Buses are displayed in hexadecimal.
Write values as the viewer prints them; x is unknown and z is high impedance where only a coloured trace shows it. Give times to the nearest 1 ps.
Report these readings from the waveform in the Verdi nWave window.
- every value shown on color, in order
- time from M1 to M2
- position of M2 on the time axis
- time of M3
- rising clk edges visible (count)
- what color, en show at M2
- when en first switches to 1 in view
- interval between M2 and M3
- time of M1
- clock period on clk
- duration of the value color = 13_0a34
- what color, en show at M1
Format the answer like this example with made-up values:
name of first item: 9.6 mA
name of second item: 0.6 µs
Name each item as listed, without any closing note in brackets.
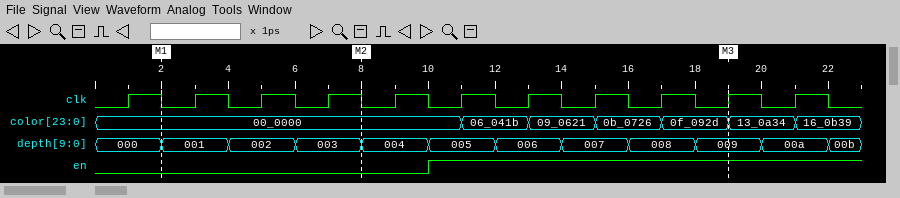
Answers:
every value shown on color, in order: 00_0000, 06_041b, 09_0621, 0b_0726, 0f_092d, 13_0a34, 16_0b39
time from M1 to M2: 6 ps
position of M2 on the time axis: 8 ps
time of M3: 19 ps
rising clk edges visible: 11
what color, en show at M2: color=00_0000, en=0
when en first switches to 1 in view: 10 ps
interval between M2 and M3: 11 ps
time of M1: 2 ps
clock period on clk: 2 ps
duration of the value color = 13_0a34: 2 ps
what color, en show at M1: color=00_0000, en=0
